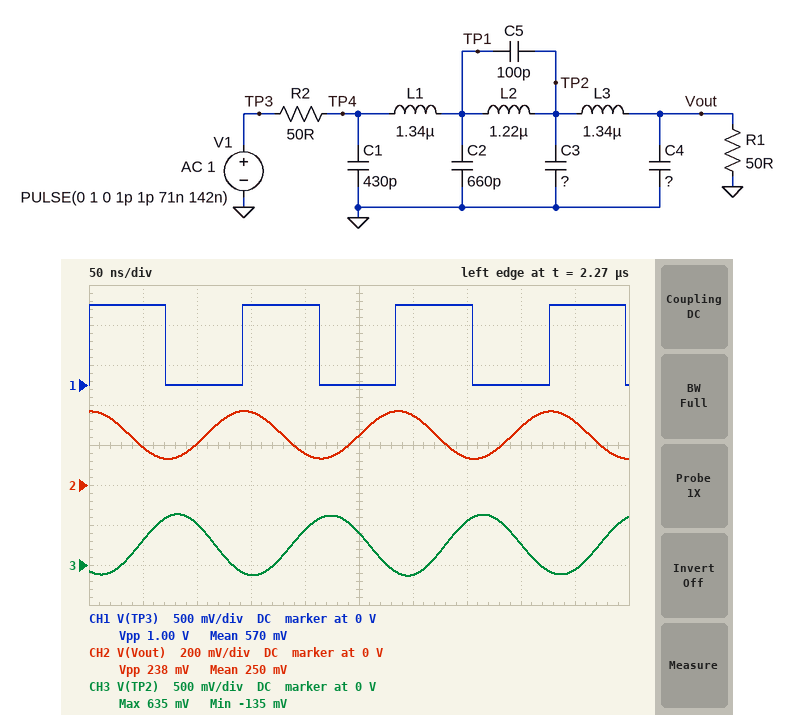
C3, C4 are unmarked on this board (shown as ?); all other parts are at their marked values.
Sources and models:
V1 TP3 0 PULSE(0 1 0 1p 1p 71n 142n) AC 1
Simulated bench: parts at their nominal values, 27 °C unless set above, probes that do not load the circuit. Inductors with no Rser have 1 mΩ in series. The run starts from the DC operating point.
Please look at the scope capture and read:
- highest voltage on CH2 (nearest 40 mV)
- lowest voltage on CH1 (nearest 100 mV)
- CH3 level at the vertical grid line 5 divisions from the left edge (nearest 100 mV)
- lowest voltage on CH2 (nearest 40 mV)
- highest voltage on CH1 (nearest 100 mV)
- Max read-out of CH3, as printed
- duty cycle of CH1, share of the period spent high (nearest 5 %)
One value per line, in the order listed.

360 mV
0 V
400 mV
120 mV
1.0 V
635 mV
50 %
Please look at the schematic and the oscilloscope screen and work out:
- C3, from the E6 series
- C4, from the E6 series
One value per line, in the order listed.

220 pF
1.5 nF
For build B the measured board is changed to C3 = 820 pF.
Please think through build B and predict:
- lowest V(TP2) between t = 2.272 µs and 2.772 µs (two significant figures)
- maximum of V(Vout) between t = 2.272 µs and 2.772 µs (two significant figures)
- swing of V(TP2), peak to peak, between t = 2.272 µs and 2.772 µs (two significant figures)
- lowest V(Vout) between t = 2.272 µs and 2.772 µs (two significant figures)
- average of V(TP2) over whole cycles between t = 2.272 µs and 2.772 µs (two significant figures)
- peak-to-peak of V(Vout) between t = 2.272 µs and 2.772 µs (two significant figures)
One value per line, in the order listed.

-410 mV
460 mV
1.3 V
42 mV
250 mV
420 mV
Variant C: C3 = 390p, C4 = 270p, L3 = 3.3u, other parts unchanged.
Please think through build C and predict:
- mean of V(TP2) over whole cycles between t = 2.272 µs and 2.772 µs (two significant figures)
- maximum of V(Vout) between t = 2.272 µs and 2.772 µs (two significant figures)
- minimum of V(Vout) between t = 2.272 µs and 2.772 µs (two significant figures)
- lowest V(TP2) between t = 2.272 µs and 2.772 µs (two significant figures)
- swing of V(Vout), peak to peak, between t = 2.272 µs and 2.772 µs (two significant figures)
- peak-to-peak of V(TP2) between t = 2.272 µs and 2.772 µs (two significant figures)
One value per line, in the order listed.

250 mV
470 mV
29 mV
-420 mV
440 mV
1.3 V
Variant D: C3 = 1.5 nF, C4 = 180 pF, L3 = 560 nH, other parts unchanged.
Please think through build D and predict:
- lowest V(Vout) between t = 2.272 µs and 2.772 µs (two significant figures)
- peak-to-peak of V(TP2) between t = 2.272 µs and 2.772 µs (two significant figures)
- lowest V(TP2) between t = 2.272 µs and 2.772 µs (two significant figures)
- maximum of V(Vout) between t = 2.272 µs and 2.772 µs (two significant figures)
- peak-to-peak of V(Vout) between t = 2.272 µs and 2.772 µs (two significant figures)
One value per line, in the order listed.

74 mV
330 mV
84 mV
430 mV
350 mV
